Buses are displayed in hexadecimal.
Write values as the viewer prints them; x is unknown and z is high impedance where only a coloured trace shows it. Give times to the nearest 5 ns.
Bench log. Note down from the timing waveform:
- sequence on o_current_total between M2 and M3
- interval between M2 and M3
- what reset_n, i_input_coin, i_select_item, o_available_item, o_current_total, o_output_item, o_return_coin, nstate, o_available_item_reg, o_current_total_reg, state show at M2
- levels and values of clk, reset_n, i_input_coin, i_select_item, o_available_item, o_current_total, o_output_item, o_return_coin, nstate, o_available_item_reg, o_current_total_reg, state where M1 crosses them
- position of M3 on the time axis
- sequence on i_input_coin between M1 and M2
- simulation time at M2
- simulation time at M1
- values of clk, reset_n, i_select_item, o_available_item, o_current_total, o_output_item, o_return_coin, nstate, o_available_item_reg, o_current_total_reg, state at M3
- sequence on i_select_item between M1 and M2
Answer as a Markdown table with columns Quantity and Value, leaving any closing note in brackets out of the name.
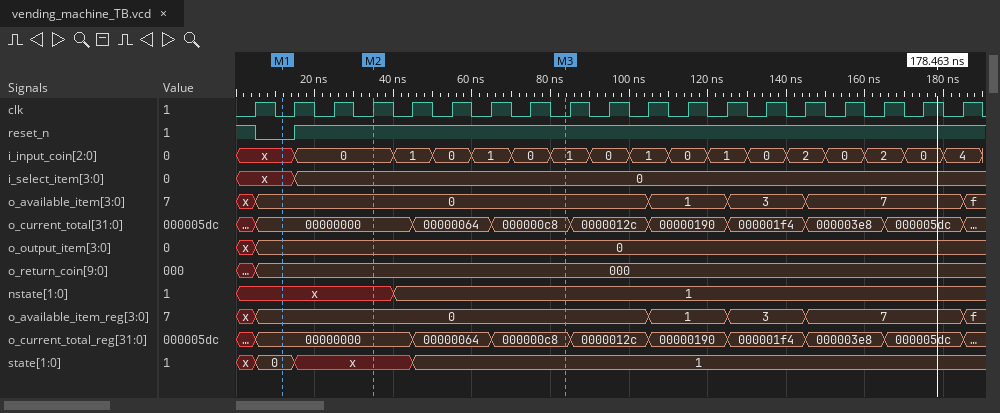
| Quantity | Value |
|---|---|
| sequence on o_current_total between M2 and M3 | 00000000, 00000064, 000000c8 |
| interval between M2 and M3 | 50 ns |
| what reset_n, i_input_coin, i_select_item, o_available_item, o_current_total, o_output_item, o_return_coin, nstate, o_available_item_reg, o_current_total_reg, state show at M2 | reset_n=1, i_input_coin=0, i_select_item=0, o_available_item=0, o_current_total=00000000, o_output_item=0, o_return_coin=000, nstate=x, o_available_item_reg=0, o_current_total_reg=00000000, state=x |
| levels and values of clk, reset_n, i_input_coin, i_select_item, o_available_item, o_current_total, o_output_item, o_return_coin, nstate, o_available_item_reg, o_current_total_reg, state where M1 crosses them | clk=0, reset_n=0, i_input_coin=x, i_select_item=x, o_available_item=0, o_current_total=00000000, o_output_item=0, o_return_coin=000, nstate=x, o_available_item_reg=0, o_current_total_reg=00000000, state=0 |
| position of M3 on the time axis | 85 ns |
| sequence on i_input_coin between M1 and M2 | x, 0 |
| simulation time at M2 | 35 ns |
| simulation time at M1 | 10 ns |
| values of clk, reset_n, i_select_item, o_available_item, o_current_total, o_output_item, o_return_coin, nstate, o_available_item_reg, o_current_total_reg, state at M3 | clk=0, reset_n=1, i_select_item=0, o_available_item=0, o_current_total=000000c8, o_output_item=0, o_return_coin=000, nstate=1, o_available_item_reg=0, o_current_total_reg=000000c8, state=1 |
| sequence on i_select_item between M1 and M2 | x, 0 |
